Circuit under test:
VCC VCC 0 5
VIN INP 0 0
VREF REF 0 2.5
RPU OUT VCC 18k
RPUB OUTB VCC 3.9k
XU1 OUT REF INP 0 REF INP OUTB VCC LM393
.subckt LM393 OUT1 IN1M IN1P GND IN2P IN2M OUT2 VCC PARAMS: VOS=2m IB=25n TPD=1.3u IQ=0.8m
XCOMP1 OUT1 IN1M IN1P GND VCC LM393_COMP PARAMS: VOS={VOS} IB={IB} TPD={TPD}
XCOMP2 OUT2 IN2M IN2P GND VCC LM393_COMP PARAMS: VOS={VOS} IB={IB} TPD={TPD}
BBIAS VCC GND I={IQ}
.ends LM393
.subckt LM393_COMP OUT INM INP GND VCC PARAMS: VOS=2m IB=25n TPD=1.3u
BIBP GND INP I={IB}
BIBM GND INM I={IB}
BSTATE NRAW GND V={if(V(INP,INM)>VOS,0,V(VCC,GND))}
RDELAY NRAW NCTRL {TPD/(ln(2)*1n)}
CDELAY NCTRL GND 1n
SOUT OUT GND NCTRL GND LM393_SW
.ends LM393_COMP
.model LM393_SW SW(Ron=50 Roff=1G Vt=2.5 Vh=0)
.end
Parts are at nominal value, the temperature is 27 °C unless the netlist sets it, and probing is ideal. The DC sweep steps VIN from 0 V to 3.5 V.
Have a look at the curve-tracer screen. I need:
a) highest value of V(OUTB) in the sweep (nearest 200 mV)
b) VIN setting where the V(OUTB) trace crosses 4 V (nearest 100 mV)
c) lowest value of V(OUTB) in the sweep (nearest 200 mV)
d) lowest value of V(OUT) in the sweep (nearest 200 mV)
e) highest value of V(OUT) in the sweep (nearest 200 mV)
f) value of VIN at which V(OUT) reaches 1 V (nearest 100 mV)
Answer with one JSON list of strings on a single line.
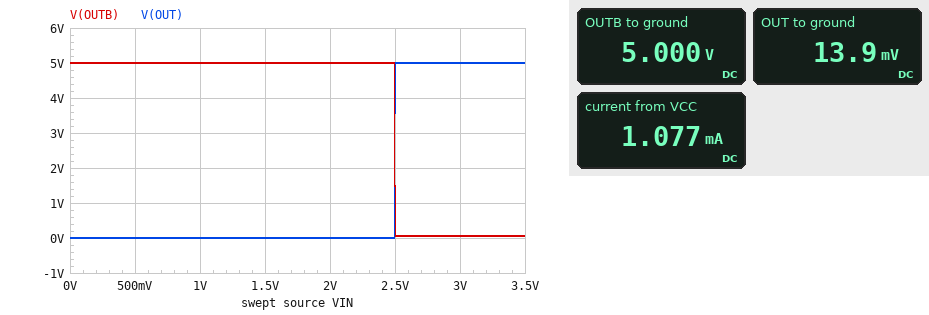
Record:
["5.0 V", "2.5 V", "0 V", "0 V", "5.0 V", "2.5 V"]
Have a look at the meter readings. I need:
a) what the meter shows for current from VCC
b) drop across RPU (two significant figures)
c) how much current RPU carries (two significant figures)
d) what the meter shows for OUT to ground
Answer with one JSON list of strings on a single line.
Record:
["1.077 mA", "5.0 V", "280 µA", "13.9 mV"]
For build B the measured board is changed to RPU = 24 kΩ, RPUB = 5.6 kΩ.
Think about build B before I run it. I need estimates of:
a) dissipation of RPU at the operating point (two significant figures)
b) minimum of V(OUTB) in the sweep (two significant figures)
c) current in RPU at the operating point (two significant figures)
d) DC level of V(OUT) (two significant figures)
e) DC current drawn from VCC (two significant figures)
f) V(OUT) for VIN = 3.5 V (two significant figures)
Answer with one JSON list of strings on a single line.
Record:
["1.0 mW", "44 mV", "210 µA", "10 mV", "1.0 mA", "5.0 V"]
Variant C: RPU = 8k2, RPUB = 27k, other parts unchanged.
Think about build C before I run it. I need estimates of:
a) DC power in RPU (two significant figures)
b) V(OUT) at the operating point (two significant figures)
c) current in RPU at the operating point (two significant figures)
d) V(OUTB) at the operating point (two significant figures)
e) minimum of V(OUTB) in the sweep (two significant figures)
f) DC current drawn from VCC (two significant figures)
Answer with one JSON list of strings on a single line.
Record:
["3.0 mW", "30 mV", "610 µA", "5.0 V", "9.2 mV", "1.4 mA"]
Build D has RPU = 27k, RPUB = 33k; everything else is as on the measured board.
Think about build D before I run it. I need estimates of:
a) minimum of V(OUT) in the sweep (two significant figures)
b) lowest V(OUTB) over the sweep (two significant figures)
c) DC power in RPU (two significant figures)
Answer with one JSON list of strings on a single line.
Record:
["9.2 mV", "7.6 mV", "920 µW"]
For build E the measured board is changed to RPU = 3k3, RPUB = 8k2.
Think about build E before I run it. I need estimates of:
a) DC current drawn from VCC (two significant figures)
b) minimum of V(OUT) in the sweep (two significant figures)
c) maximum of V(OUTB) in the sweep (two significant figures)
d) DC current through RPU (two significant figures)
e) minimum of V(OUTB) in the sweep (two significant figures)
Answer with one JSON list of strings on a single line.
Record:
["2.3 mA", "75 mV", "5.0 V", "1.5 mA", "30 mV"]
